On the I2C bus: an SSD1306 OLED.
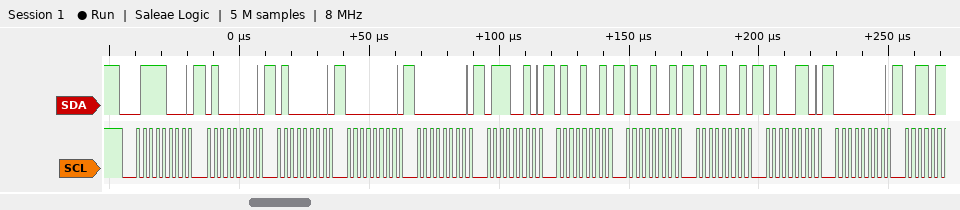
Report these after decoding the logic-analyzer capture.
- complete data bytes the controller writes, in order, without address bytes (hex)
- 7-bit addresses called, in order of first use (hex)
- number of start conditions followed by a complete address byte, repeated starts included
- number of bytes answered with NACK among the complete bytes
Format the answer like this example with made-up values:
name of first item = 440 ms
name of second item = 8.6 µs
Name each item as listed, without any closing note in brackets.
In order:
complete data bytes the controller writes, in order, without address bytes = 40 40 00 00 72 49 49 49 46 00
7-bit addresses called, in order of first use = 0x3C
number of start conditions followed by a complete address byte, repeated starts included = 1
number of bytes answered with NACK among the complete bytes = 0
